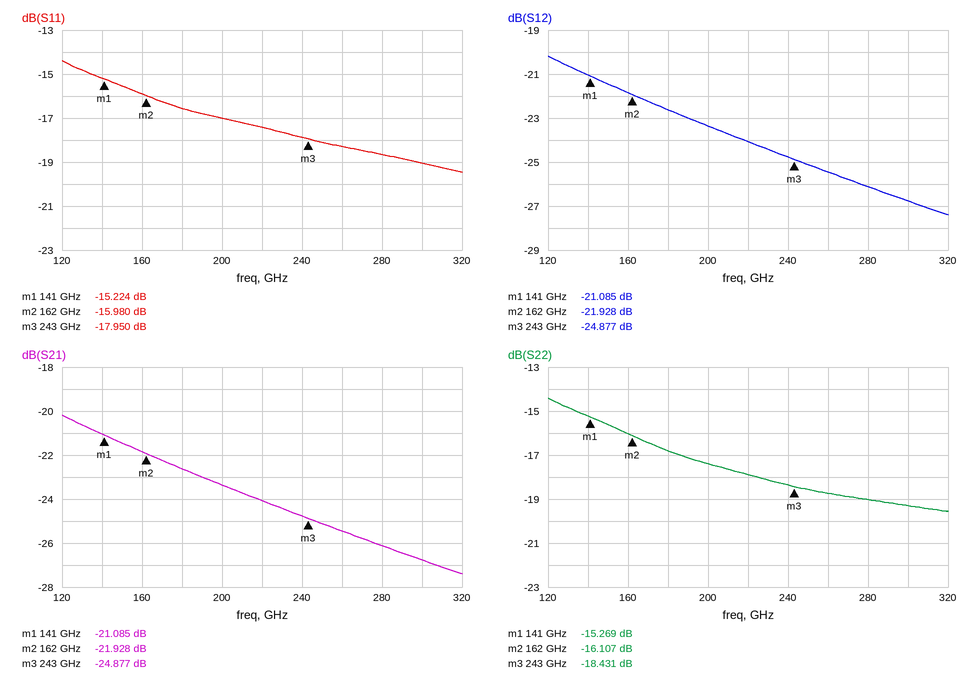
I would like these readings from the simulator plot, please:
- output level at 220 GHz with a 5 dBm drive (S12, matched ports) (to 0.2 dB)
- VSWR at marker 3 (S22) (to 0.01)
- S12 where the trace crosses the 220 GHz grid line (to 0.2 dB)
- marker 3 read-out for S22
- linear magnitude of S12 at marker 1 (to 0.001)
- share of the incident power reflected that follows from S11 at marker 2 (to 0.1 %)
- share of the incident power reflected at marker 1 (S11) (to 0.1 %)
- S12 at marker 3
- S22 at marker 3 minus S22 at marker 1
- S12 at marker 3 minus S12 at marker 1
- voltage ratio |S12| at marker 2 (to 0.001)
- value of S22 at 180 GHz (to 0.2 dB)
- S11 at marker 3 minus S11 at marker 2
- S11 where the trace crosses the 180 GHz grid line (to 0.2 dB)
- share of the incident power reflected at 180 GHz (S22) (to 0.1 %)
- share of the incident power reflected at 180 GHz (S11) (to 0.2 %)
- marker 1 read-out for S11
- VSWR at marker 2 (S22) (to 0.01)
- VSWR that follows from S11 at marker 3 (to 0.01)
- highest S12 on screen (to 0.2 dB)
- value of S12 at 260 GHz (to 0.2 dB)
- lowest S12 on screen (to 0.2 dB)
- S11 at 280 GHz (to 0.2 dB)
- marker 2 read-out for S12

-19.0 dBm
1.27
-24.0 dB
-18.431 dB
0.088
2.5 %
3.0 %
-24.877 dB
-3.162 dB
-3.792 dB
0.080
-16.8 dB
-1.970 dB
-16.6 dB
2.1 %
2.2 %
-15.224 dB
1.37
1.29
-20.2 dB
-25.4 dB
-27.4 dB
-18.6 dB
-21.928 dB
